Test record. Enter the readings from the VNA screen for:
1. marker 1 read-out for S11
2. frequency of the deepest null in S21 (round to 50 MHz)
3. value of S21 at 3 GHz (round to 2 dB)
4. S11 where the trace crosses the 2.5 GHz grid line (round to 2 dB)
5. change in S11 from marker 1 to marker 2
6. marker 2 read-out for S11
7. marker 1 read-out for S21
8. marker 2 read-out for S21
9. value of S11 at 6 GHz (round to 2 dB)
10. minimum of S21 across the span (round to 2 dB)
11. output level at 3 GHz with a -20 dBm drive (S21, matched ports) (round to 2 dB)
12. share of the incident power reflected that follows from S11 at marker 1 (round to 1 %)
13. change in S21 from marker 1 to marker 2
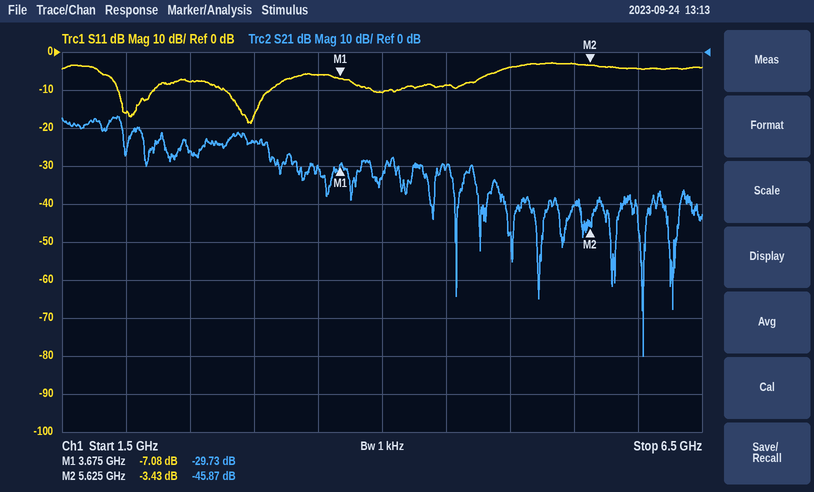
-7.08 dB
6.05 GHz
-24 dB
-8 dB
3.65 dB
-3.43 dB
-29.73 dB
-45.87 dB
-4 dB
-80 dB
-44 dBm
20 %
-16.14 dB
